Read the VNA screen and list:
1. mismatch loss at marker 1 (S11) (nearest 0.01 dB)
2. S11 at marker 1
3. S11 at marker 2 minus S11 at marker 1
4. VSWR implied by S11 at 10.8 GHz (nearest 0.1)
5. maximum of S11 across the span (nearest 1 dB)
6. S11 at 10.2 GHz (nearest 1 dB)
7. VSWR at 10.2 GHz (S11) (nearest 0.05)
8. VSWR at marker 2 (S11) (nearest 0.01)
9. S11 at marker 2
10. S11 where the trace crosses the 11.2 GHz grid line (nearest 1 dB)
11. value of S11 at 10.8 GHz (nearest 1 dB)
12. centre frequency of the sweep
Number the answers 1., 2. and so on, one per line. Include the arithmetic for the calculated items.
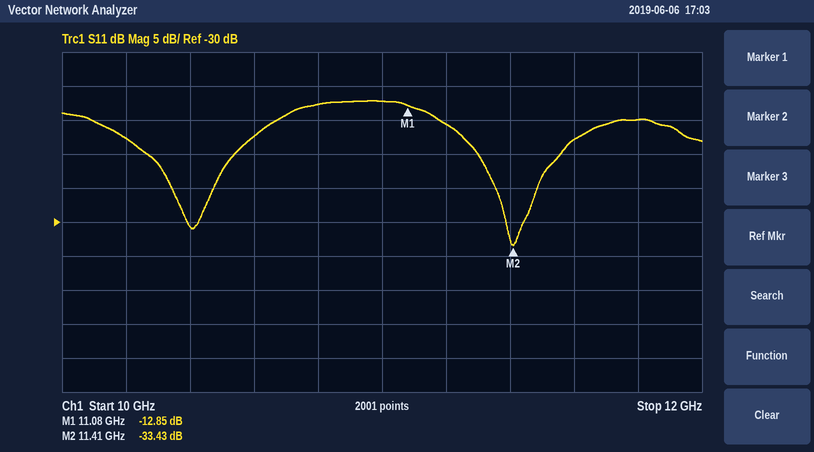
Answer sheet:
1. −10 log10(1 − 10^(-12.85/10)) ≈ 0.23 dB
2. -12.85 dB
3. -33.43 − (-12.85) = -20.58 dB
4. |Γ| = 10^(-13/20) = 0.2239; VSWR = (1 + 0.2239)/(1 − 0.2239) ≈ 1.6
5. -12 dB
6. -18 dB
7. |Γ| = 10^(-18/20) = 0.1259; VSWR = (1 + 0.1259)/(1 − 0.1259) ≈ 1.29, so 1.30 to the nearest 0.05
8. (1 + 0.0213)/(1 − 0.0213) ≈ 1.04
9. -33.43 dB
10. -16 dB
11. -13 dB
12. 11 GHz
